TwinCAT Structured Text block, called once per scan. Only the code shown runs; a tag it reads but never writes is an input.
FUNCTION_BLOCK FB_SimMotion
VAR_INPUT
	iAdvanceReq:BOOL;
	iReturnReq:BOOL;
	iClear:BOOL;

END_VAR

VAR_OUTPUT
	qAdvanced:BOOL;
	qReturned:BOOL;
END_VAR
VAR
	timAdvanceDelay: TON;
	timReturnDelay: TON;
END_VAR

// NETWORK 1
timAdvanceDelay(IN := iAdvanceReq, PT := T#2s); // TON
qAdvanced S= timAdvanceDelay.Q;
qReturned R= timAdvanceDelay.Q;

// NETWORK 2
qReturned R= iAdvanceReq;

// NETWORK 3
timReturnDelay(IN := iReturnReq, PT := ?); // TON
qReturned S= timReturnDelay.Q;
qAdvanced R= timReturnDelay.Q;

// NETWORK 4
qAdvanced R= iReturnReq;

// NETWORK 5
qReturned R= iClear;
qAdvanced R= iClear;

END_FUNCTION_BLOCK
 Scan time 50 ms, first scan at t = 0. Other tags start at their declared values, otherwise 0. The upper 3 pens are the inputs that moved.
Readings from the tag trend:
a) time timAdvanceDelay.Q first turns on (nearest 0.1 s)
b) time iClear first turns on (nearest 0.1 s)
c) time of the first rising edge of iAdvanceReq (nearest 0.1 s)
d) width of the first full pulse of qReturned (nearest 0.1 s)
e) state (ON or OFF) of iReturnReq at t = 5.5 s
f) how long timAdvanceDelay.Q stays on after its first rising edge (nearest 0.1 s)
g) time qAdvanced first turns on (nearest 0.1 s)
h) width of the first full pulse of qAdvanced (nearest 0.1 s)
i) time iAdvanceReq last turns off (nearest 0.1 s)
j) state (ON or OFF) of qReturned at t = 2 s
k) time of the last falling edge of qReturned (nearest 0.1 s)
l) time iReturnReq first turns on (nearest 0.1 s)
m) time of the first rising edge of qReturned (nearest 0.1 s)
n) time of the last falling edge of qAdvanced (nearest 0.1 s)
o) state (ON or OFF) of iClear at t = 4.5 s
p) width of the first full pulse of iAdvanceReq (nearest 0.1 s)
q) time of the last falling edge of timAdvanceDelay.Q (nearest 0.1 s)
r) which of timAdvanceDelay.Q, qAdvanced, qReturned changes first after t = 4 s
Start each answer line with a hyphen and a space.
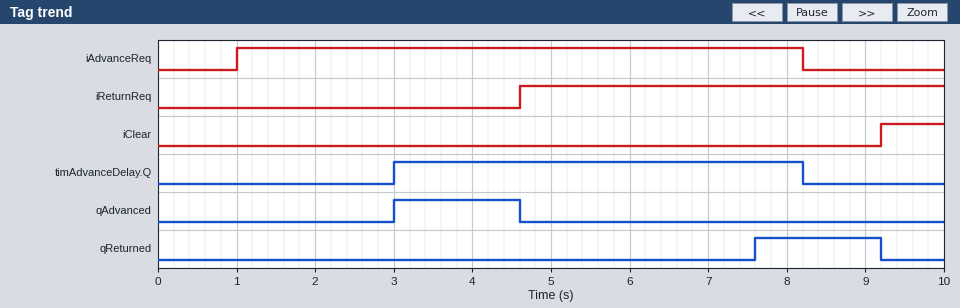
- 3.0 s
- 9.2 s
- 1.0 s
- 1.6 s
- ON
- 5.2 s
- 3.0 s
- 1.6 s
- 8.2 s
- OFF
- 9.2 s
- 4.6 s
- 7.6 s
- 4.6 s
- OFF
- 7.2 s
- 8.2 s
- qAdvanced
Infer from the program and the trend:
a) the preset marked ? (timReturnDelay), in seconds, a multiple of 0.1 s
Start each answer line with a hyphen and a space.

- 3.0 s
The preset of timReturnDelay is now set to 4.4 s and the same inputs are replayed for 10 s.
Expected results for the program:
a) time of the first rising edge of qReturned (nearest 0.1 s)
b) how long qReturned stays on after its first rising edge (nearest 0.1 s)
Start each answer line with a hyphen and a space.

- 9.0 s
- 0.2 s
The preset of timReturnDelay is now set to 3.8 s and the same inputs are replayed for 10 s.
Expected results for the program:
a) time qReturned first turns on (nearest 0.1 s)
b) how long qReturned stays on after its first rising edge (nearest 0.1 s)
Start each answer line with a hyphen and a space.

- 8.4 s
- 0.8 s
